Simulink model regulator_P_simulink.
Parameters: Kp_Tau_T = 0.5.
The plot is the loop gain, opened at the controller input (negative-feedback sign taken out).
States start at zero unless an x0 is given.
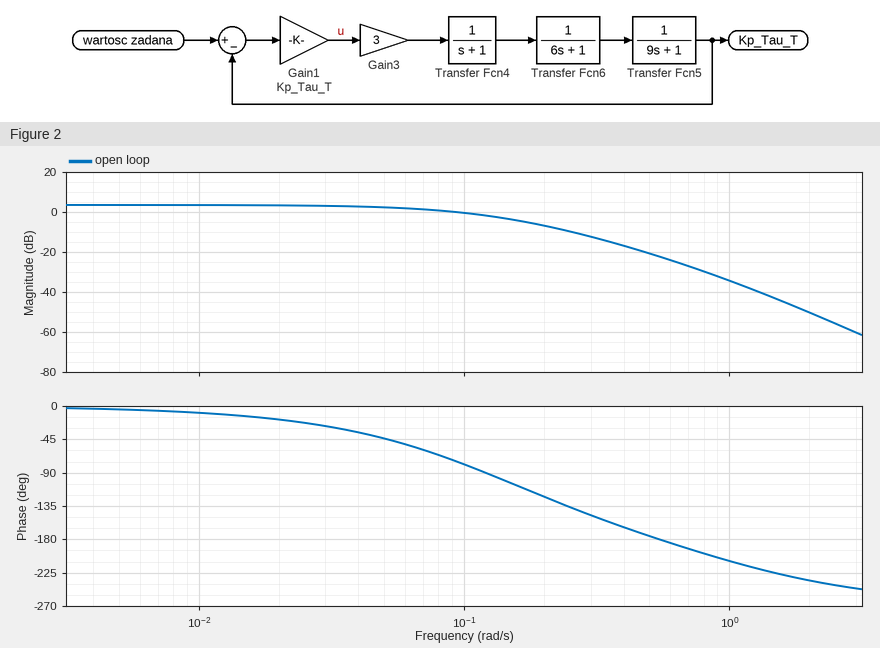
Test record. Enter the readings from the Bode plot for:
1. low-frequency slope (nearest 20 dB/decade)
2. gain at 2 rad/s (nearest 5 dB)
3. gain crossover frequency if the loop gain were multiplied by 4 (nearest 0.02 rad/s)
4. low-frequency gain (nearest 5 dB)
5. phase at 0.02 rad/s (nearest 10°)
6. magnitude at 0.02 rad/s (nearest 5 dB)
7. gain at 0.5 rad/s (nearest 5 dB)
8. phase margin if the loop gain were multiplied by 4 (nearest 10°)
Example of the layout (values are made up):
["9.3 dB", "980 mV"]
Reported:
["0 dB/decade", "-50 dB", "0.30 rad/s", "5 dB", "-20°", "5 dB", "-20 dB", "30°"]
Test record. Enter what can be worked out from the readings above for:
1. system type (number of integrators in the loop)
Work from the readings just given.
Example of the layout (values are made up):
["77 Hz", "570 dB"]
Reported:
["0"]
